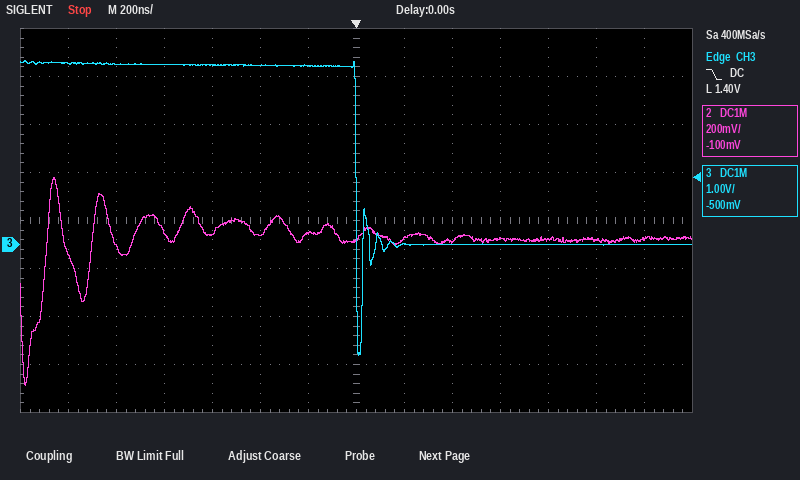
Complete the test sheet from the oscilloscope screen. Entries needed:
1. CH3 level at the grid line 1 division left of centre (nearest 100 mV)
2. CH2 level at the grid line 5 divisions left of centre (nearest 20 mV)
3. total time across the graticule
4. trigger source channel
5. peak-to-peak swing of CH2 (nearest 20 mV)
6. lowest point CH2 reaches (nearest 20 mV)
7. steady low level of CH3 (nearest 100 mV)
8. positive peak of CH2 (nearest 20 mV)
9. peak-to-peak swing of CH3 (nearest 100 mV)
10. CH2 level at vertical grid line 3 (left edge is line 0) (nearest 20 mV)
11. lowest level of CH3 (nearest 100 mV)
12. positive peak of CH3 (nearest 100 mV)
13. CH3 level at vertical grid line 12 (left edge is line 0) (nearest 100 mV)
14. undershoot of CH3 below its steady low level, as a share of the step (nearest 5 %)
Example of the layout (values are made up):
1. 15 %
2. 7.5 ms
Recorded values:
1. 3.7 V
2. 0 mV
3. 2.8 µs
4. CH3
5. 860 mV
6. -580 mV
7. 0.0 V
8. 280 mV
9. 6.1 V
10. 60 mV
11. -2.3 V
12. 3.8 V
13. 0.0 V
14. 60 %
